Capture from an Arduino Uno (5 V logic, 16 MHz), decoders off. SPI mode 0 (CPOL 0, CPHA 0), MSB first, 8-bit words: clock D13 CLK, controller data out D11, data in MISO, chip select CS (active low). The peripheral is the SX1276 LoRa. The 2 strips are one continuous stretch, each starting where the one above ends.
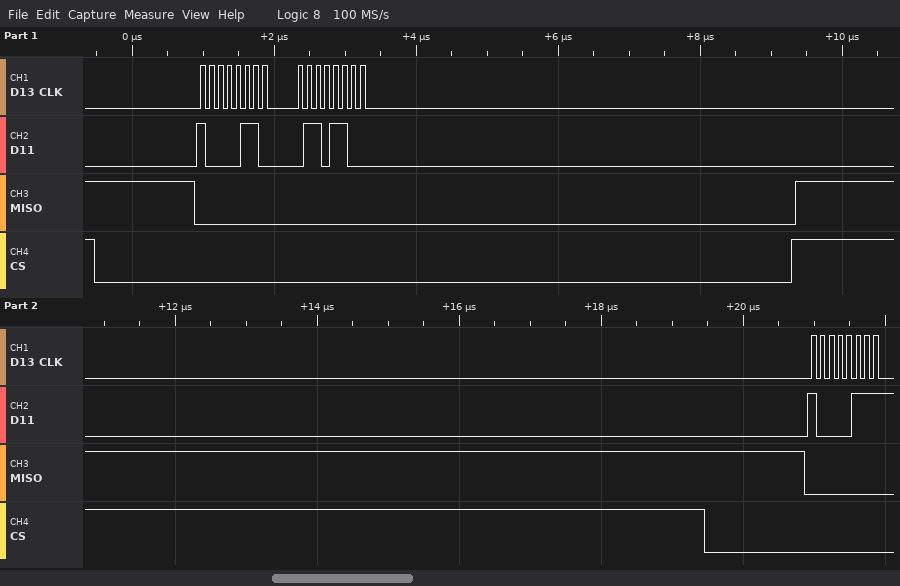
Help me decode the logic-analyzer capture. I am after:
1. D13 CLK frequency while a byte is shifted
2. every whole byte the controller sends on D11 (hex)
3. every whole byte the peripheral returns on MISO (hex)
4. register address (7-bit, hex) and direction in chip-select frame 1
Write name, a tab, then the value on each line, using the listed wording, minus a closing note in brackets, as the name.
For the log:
D13 CLK frequency while a byte is shifted	8 MHz
every whole byte the controller sends on D11	86 6C 87
every whole byte the peripheral returns on MISO	00 00 00
register address (7-bit, hex) and direction in chip-select frame 1	0x06 write
